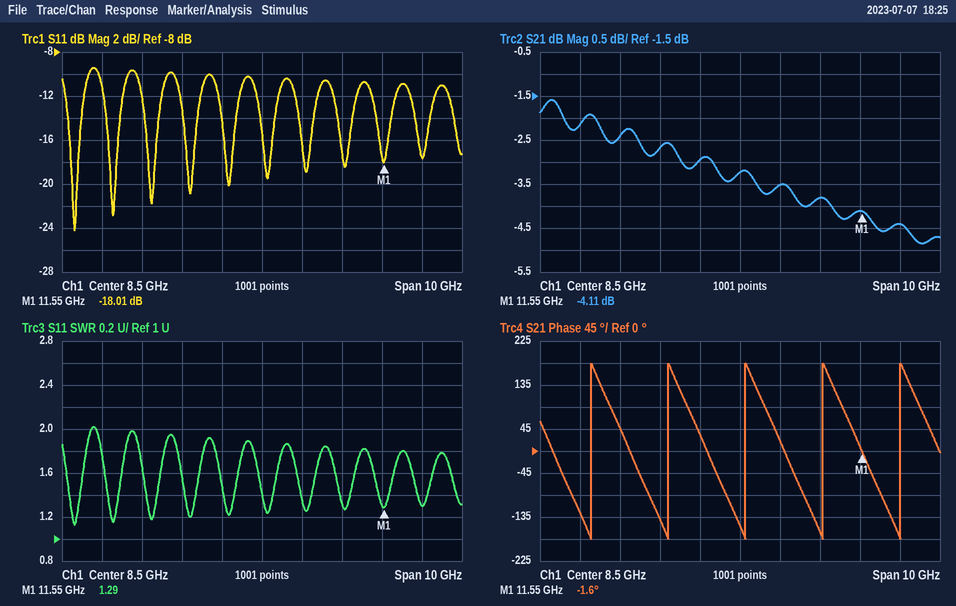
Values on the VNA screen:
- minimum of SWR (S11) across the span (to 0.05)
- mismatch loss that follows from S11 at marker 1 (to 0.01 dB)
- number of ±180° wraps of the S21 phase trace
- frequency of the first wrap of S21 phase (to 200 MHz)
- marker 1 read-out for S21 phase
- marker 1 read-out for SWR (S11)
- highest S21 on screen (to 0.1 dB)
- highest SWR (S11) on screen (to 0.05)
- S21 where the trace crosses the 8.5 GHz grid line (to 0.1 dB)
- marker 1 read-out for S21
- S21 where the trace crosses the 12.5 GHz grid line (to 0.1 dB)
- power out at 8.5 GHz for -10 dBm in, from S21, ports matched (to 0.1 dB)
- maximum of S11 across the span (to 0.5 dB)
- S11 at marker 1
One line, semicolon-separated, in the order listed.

1.15; 0.07 dB; 5; 4.8 GHz; -1.6°; 1.29; -1.6 dB; 2.00; -3.2 dB; -4.11 dB; -4.4 dB; -13.2 dBm; -9.5 dB; -18.01 dB
